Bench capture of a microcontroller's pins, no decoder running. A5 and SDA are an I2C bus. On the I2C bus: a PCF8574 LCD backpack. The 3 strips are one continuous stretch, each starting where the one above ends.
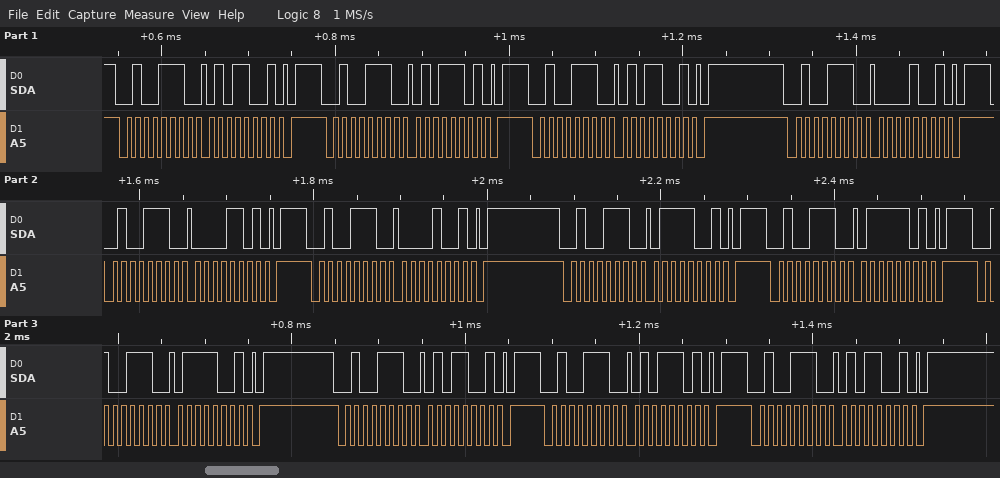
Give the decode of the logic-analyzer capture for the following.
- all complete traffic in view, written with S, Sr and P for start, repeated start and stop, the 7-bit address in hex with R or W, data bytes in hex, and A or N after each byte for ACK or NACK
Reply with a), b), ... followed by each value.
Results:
a) S 27W A 59 A P S 27W A 5D A P S 27W A 59 A P S 27W A 09 A P S 27W A 0D A P S 27W A 09 A P S 27W A 79 A P S 27W A 7D A P S 27W A 79 A P S 27W A 59 A P S 27W A 5D A P S 27W A 59 A P
